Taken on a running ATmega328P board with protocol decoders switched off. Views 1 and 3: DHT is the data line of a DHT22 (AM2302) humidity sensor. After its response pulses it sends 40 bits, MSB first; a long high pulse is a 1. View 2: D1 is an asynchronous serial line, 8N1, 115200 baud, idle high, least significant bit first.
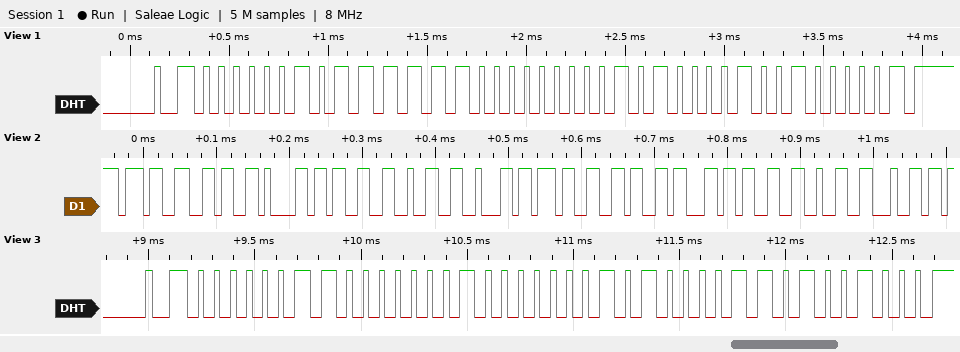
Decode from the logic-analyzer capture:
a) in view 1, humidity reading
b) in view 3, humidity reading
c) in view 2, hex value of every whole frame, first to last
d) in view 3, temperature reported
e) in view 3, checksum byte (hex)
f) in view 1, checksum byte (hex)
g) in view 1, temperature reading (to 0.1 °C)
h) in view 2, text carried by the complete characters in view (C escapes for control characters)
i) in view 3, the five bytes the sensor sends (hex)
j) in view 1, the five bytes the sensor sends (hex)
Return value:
76.4 %
76.9 %
37 36 61 33 32 62 37 36 63 33 32 64
32.3 °C
0x48
0x41
32.2 °C
"76a32b76c32d"
03 01 01 43 48
02 FC 01 42 41
